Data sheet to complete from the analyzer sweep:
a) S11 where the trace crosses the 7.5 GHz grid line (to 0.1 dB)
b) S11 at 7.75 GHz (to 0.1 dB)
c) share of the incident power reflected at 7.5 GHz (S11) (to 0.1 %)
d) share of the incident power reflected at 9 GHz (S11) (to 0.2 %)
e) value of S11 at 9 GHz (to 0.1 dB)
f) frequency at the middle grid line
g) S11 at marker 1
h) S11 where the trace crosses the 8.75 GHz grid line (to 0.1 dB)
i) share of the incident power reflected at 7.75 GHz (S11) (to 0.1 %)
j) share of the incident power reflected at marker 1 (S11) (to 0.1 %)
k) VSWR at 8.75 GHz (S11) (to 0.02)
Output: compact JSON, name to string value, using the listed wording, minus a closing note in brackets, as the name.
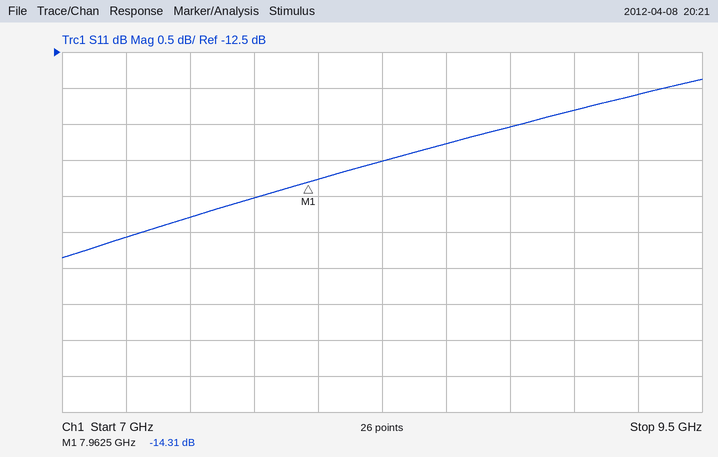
{"S11 where the trace crosses the 7.5 GHz grid line": "-14.8 dB", "S11 at 7.75 GHz": "-14.5 dB", "share of the incident power reflected at 7.5 GHz (S11)": "3.3 %", "share of the incident power reflected at 9 GHz (S11)": "4.6 %", "value of S11 at 9 GHz": "-13.3 dB", "frequency at the middle grid line": "8.25 GHz", "S11 at marker 1": "-14.31 dB", "S11 where the trace crosses the 8.75 GHz grid line": "-13.5 dB", "share of the incident power reflected at 7.75 GHz (S11)": "3.5 %", "share of the incident power reflected at marker 1 (S11)": "3.7 %", "VSWR at 8.75 GHz (S11)": "1.54"}
